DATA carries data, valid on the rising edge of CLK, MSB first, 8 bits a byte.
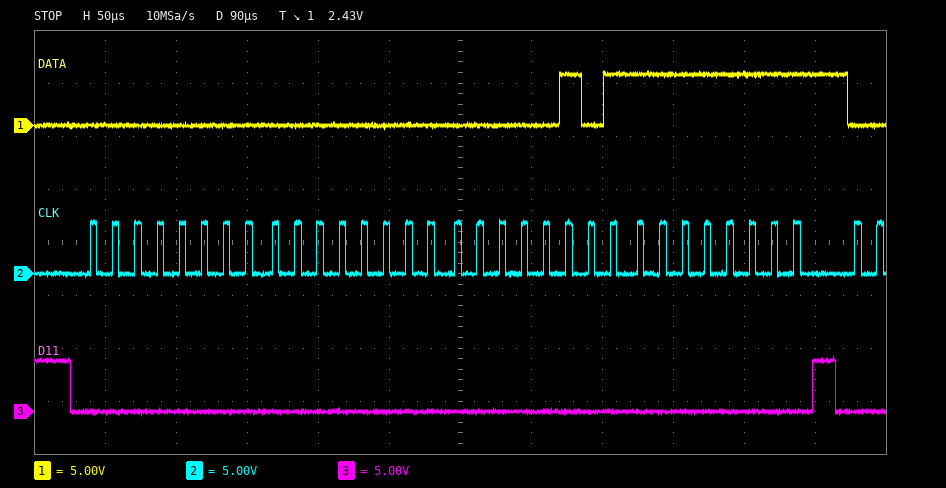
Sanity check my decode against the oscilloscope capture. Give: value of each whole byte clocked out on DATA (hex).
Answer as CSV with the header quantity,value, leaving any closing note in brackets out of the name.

quantity,value
value of each whole byte clocked out on DATA,0x00 0x00 0x05 0xFF
